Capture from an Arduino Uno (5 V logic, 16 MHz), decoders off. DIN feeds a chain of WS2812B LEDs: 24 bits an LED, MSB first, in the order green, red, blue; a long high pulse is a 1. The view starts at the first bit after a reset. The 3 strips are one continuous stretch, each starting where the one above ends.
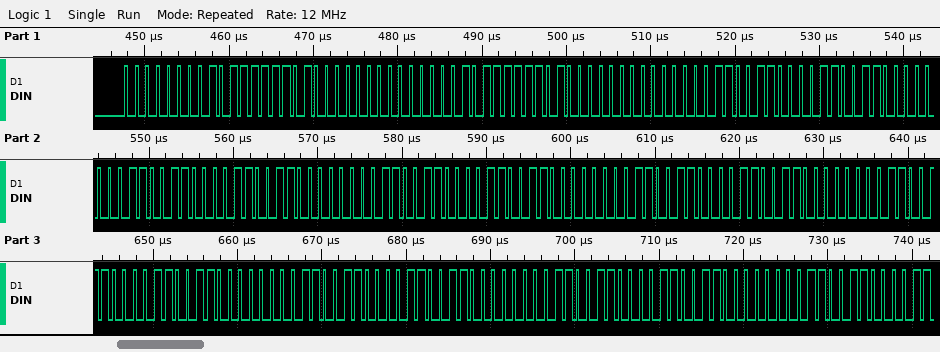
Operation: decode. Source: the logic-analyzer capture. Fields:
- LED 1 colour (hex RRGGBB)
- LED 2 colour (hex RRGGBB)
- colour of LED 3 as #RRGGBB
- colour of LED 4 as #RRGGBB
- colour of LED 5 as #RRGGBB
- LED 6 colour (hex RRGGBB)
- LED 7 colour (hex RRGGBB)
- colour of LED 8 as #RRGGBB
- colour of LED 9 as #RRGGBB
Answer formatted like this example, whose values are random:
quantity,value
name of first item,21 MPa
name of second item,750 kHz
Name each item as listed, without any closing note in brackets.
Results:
quantity,value
LED 1 colour,#BF0040
LED 2 colour,#BF0040
colour of LED 3 as #RRGGBB,#CC0033
colour of LED 4 as #RRGGBB,#CC0033
colour of LED 5 as #RRGGBB,#CC0033
LED 6 colour,#CC0033
LED 7 colour,#CC0033
colour of LED 8 as #RRGGBB,#CC0033
colour of LED 9 as #RRGGBB,#CC0033
